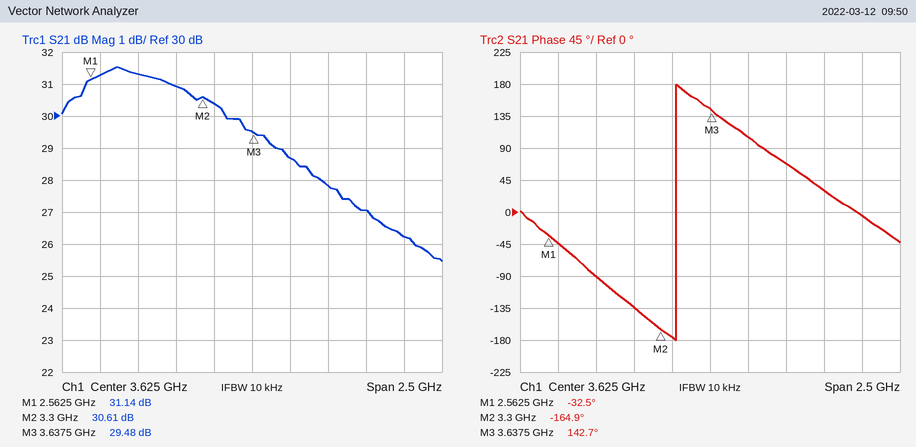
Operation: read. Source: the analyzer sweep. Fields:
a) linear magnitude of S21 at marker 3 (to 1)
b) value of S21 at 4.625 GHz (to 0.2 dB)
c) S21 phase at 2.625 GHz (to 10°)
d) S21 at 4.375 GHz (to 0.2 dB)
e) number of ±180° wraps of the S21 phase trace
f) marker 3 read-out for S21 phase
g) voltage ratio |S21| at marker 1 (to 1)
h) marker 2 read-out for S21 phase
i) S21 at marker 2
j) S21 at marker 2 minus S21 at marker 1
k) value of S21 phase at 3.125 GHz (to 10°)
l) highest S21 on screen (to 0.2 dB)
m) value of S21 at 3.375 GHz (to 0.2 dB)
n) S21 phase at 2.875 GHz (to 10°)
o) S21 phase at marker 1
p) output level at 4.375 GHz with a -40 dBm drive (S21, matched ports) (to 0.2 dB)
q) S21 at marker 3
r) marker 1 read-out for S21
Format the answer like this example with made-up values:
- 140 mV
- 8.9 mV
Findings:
- 30
- 26.2 dB
- -40°
- 27.0 dB
- 1
- 142.7°
- 36
- -164.9°
- 30.61 dB
- -0.53 dB
- -130°
- 31.6 dB
- 30.4 dB
- -90°
- -32.5°
- -13.0 dBm
- 29.48 dB
- 31.14 dB
